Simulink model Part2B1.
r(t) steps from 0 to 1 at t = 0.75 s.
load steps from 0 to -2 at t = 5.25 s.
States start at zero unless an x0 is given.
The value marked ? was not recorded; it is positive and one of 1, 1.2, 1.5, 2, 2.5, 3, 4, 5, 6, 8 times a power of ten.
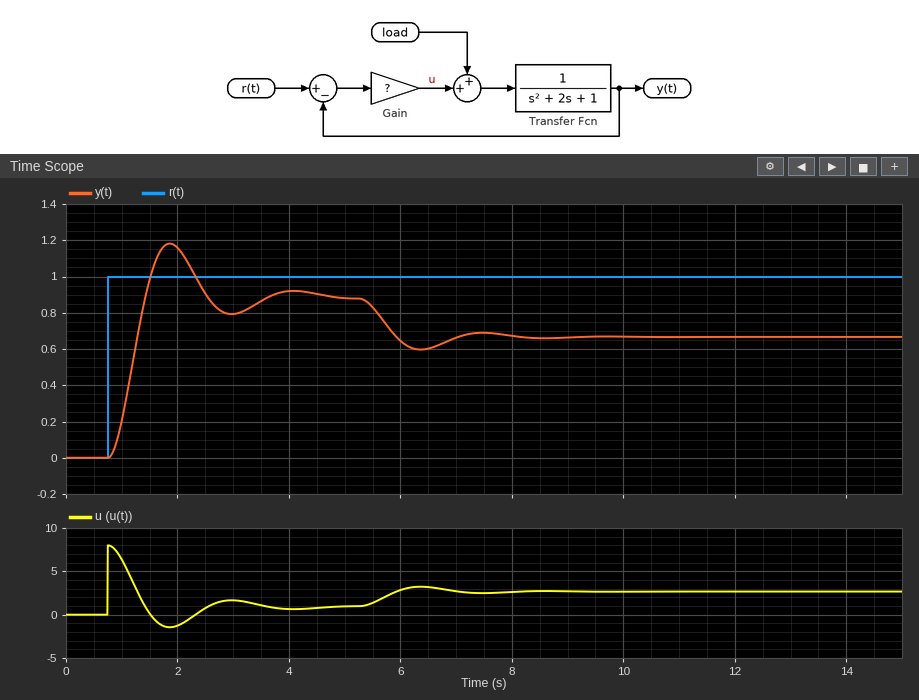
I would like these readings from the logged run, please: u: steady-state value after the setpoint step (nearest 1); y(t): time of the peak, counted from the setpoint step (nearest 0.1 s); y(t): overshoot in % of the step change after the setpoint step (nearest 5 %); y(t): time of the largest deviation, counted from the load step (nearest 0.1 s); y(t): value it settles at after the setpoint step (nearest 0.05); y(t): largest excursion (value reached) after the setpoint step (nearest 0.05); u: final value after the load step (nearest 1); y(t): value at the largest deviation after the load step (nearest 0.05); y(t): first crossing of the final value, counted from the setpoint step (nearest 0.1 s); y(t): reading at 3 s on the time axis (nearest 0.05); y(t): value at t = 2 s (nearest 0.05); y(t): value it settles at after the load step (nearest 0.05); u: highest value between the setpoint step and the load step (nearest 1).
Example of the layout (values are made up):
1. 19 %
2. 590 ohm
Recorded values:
1. 1
2. 1.1 s
3. 35 %
4. 1.1 s
5. 0.90
6. 1.20
7. 3
8. 0.60
9. 0.7 s
10. 0.80
11. 1.15
12. 0.65
13. 8
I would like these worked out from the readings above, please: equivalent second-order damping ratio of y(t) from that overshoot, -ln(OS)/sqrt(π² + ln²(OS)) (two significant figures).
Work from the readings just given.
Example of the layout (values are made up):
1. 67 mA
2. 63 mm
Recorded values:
1. 0.32
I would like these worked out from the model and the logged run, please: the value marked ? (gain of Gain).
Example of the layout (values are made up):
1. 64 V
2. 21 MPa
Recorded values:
1. 8
